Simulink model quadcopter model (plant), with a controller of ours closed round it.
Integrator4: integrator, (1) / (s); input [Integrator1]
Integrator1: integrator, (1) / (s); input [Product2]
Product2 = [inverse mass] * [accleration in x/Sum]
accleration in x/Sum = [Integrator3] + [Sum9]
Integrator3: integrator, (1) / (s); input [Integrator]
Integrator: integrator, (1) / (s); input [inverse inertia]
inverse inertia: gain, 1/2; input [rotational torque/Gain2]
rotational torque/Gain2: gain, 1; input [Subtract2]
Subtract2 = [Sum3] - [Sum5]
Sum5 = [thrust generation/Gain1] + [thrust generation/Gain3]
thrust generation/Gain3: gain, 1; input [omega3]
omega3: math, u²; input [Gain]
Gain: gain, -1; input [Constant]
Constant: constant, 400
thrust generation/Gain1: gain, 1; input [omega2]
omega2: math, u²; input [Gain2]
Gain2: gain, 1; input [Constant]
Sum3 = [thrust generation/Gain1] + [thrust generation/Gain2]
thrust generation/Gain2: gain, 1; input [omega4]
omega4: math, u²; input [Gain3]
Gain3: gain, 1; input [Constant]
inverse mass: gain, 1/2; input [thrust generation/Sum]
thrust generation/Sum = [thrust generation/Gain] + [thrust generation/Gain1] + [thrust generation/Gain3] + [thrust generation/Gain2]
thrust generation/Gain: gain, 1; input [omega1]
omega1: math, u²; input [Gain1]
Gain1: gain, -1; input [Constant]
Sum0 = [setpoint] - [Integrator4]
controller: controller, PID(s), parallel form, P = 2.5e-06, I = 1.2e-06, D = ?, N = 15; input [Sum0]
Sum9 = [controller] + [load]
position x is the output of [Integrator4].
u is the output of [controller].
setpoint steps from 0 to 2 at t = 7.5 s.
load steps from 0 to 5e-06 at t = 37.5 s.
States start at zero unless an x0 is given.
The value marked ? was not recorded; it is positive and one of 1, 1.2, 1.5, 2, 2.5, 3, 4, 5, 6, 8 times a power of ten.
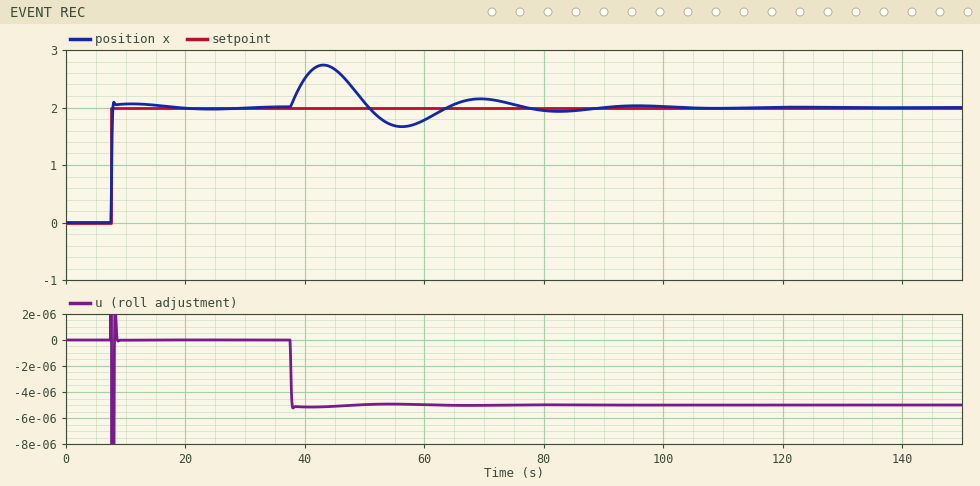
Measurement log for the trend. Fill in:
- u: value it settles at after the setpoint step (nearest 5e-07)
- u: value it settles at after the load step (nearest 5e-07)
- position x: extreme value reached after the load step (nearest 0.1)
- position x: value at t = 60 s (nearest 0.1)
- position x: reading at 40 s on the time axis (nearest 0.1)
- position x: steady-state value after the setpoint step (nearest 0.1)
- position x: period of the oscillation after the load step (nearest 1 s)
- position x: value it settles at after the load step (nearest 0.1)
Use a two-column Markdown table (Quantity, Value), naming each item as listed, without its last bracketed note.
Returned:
| Quantity | Value |
|---|---|
| u: value it settles at after the setpoint step | 0.0000000 |
| u: value it settles at after the load step | -0.0000050 |
| position x: extreme value reached after the load step | 2.7 |
| position x: value at t = 60 s | 1.8 |
| position x: reading at 40 s on the time axis | 2.5 |
| position x: steady-state value after the setpoint step | 2.0 |
| position x: period of the oscillation after the load step | 26 s |
| position x: value it settles at after the load step | 2.0 |
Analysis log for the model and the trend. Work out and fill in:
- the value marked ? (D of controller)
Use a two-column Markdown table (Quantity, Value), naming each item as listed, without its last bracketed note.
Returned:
| Quantity | Value |
|---|---|
| the value marked ? | 2e-05 |
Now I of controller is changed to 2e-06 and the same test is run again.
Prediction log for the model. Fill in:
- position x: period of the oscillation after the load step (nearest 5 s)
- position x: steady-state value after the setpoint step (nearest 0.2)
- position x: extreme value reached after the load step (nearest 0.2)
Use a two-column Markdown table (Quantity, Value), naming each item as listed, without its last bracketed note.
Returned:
| Quantity | Value |
|---|---|
| position x: period of the oscillation after the load step | 20 s |
| position x: steady-state value after the setpoint step | 2.0 |
| position x: extreme value reached after the load step | 2.6 |
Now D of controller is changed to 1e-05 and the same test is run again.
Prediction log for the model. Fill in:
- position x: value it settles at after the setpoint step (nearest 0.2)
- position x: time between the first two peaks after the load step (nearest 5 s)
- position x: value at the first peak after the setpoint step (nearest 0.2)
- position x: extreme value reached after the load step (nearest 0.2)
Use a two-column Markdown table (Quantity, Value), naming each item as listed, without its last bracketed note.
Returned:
| Quantity | Value |
|---|---|
| position x: value it settles at after the setpoint step | 2.0 |
| position x: time between the first two peaks after the load step | 20 s |
| position x: value at the first peak after the setpoint step | 2.2 |
| position x: extreme value reached after the load step | 3.0 |
